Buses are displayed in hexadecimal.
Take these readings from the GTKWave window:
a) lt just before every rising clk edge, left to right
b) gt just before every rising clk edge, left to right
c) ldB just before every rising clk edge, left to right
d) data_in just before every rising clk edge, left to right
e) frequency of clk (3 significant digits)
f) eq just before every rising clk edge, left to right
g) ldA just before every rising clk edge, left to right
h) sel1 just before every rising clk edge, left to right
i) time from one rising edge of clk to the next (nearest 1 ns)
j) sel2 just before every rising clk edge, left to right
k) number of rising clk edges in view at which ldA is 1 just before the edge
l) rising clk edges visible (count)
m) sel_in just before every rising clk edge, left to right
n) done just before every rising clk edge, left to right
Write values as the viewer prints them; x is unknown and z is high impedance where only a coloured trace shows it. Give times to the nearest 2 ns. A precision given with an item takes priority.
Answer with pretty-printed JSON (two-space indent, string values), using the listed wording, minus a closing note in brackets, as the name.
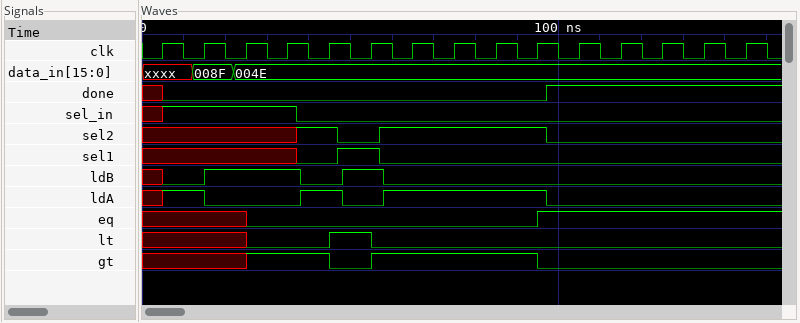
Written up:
{
  "lt just before every rising clk edge, left to right": "x x x 0 0 1 0 0 0 0 0 0 0 0 0",
  "gt just before every rising clk edge, left to right": "x x x 1 1 0 1 1 1 1 0 0 0 0 0",
  "ldB just before every rising clk edge, left to right": "x 0 1 1 0 1 0 0 0 0 0 0 0 0 0",
  "data_in just before every rising clk edge, left to right": "xxxx, 008F, 004E, 004E, 004E, 004E, 004E, 004E, 004E, 004E, 004E, 004E, 004E, 004E, 004E",
  "frequency of clk": "100 MHz",
  "eq just before every rising clk edge, left to right": "x x x 0 0 0 0 0 0 0 1 1 1 1 1",
  "ldA just before every rising clk edge, left to right": "x 1 0 0 1 0 1 1 1 1 0 0 0 0 0",
  "sel1 just before every rising clk edge, left to right": "x x x x 0 1 0 0 0 0 0 0 0 0 0",
  "time from one rising edge of clk to the next": "10 ns",
  "sel2 just before every rising clk edge, left to right": "x x x x 1 0 1 1 1 1 0 0 0 0 0",
  "number of rising clk edges in view at which ldA is 1 just before the edge": "6",
  "rising clk edges visible": "15",
  "sel_in just before every rising clk edge, left to right": "x 1 1 1 0 0 0 0 0 0 0 0 0 0 0",
  "done just before every rising clk edge, left to right": "x 0 0 0 0 0 0 0 0 0 1 1 1 1 1"
}
